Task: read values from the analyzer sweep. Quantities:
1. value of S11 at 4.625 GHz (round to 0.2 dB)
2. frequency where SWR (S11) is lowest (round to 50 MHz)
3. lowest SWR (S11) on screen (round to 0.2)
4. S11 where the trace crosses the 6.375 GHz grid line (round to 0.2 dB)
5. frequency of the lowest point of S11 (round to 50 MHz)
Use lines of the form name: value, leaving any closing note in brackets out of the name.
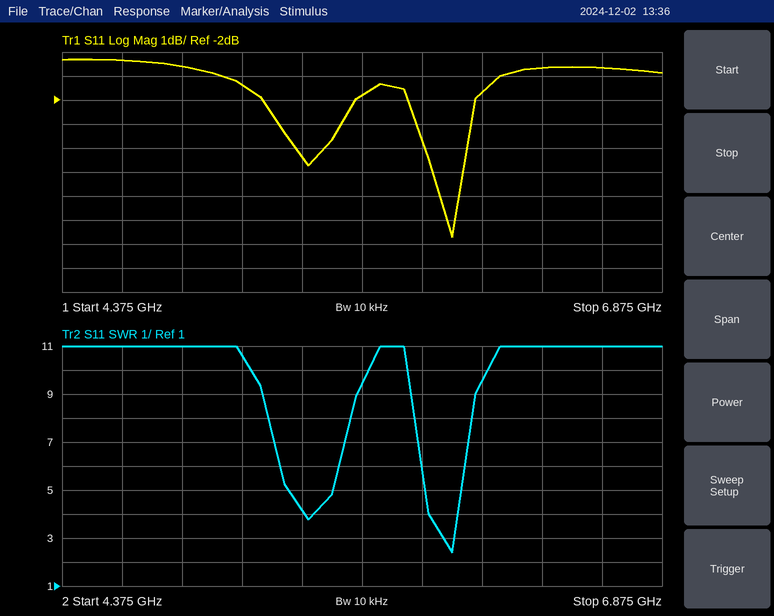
value of S11 at 4.625 GHz: -0.4 dB
frequency where SWR (S11) is lowest: 6.00 GHz
lowest SWR (S11) on screen: 2.4
S11 where the trace crosses the 6.375 GHz grid line: -0.6 dB
frequency of the lowest point of S11: 6.00 GHz
